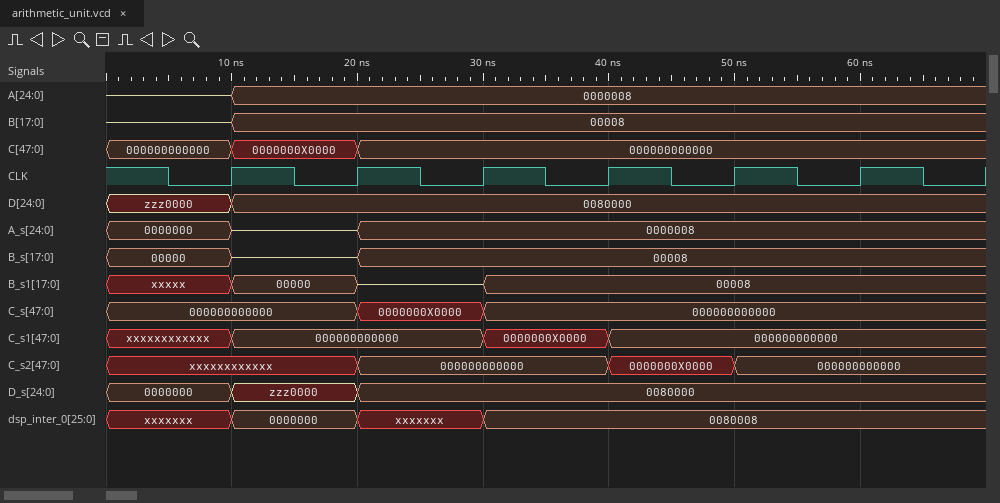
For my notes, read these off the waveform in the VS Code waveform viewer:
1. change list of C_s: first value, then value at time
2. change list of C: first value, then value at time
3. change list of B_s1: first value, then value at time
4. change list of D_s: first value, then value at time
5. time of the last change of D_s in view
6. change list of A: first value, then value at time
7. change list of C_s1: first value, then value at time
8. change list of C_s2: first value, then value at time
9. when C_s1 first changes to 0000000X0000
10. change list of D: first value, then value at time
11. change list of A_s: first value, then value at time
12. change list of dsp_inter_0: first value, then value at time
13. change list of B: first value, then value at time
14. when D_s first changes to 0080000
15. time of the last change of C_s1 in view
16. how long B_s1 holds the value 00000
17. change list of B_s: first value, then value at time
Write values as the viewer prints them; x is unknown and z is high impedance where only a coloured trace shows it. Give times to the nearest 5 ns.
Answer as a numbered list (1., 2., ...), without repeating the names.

1. 000000000000, 0000000X0000 at 20 ns, 000000000000 at 30 ns
2. 000000000000, 0000000X0000 at 10 ns, 000000000000 at 20 ns
3. xxxxx, 00000 at 10 ns, z at 20 ns, 00008 at 30 ns
4. 0000000, zzz0000 at 10 ns, 0080000 at 20 ns
5. 20 ns
6. z, 0000008 at 10 ns
7. xxxxxxxxxxxx, 000000000000 at 10 ns, 0000000X0000 at 30 ns, 000000000000 at 40 ns
8. xxxxxxxxxxxx, 000000000000 at 20 ns, 0000000X0000 at 40 ns, 000000000000 at 50 ns
9. 30 ns
10. zzz0000, 0080000 at 10 ns
11. 0000000, z at 10 ns, 0000008 at 20 ns
12. xxxxxxx, 0000000 at 10 ns, xxxxxxx at 20 ns, 0080008 at 30 ns
13. z, 00008 at 10 ns
14. 20 ns
15. 40 ns
16. 10 ns
17. 00000, z at 10 ns, 00008 at 20 ns
